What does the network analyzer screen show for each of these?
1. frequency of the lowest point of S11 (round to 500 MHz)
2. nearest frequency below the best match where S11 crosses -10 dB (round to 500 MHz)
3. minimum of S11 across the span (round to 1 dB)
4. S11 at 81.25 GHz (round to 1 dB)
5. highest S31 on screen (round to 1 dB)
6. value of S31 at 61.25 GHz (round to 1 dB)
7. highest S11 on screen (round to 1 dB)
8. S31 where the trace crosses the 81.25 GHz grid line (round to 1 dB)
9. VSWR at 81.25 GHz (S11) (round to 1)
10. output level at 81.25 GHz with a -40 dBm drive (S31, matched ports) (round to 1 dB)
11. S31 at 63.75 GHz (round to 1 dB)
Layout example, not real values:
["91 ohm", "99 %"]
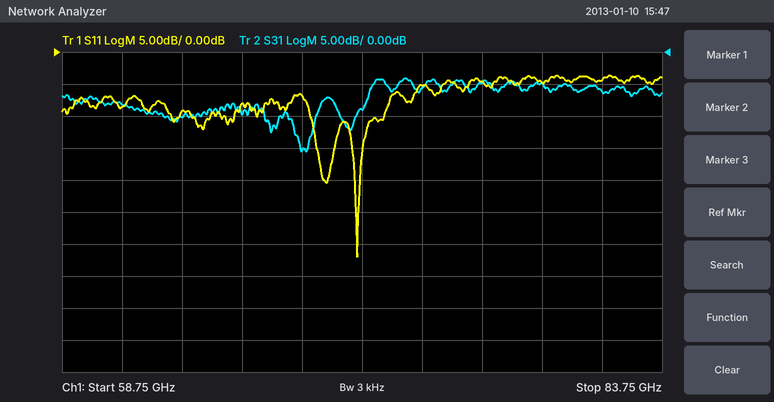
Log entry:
["71.0 GHz", "69.0 GHz", "-32 dB", "-4 dB", "-4 dB", "-8 dB", "-4 dB", "-6 dB", "4", "-46 dBm", "-10 dB"]
